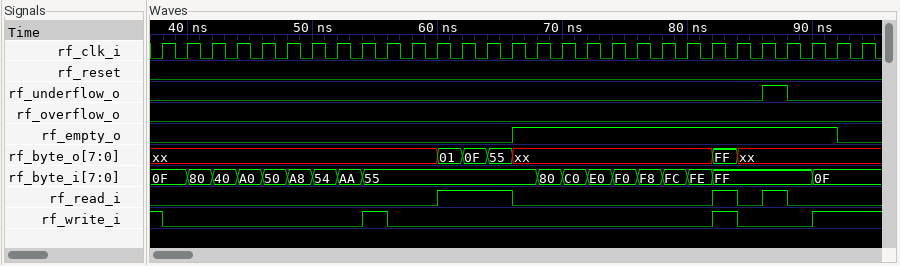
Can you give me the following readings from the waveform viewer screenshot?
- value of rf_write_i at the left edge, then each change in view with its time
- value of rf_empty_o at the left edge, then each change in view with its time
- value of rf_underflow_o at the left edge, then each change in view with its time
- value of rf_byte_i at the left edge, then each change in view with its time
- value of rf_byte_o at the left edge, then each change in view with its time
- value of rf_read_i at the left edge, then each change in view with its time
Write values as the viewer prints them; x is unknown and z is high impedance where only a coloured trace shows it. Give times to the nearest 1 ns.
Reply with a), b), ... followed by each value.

a) 1, 0 at 38 ns, 1 at 54 ns, 0 at 56 ns, 1 at 82 ns, 0 at 84 ns, 1 at 90 ns
b) 0, 1 at 66 ns, 0 at 92 ns
c) 0, 1 at 86 ns, 0 at 88 ns
d) 0F, 80 at 40 ns, 40 at 42 ns, A0 at 44 ns, 50 at 46 ns, A8 at 48 ns, 54 at 50 ns, AA at 52 ns, 55 at 54 ns, 80 at 68 ns, C0 at 70 ns, E0 at 72 ns, F0 at 74 ns, F8 at 76 ns, FC at 78 ns, FE at 80 ns, FF at 82 ns, 0F at 90 ns
e) xx, 01 at 60 ns, 0F at 62 ns, 55 at 64 ns, xx at 66 ns, FF at 82 ns, xx at 84 ns
f) 0, 1 at 60 ns, 0 at 66 ns, 1 at 82 ns, 0 at 84 ns, 1 at 86 ns, 0 at 88 ns
